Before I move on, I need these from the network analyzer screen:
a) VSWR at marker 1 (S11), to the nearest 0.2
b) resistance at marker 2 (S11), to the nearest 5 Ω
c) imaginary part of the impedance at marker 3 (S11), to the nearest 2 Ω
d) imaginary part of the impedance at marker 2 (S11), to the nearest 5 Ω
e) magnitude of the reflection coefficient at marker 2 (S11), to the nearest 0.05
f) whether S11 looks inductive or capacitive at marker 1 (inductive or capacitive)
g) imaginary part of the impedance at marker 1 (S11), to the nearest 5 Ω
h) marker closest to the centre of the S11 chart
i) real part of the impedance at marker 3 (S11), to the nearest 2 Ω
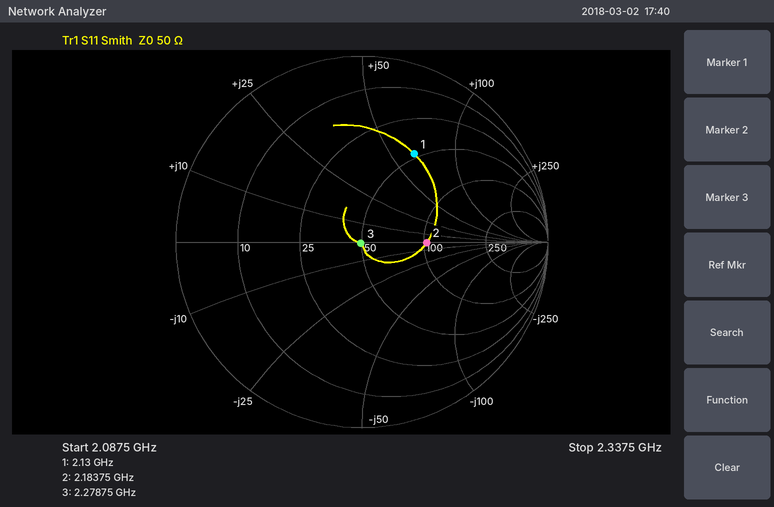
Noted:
3.4
105 Ω
0 Ω
0 Ω
0.35
inductive
+65 Ω
marker 3
50 Ω
